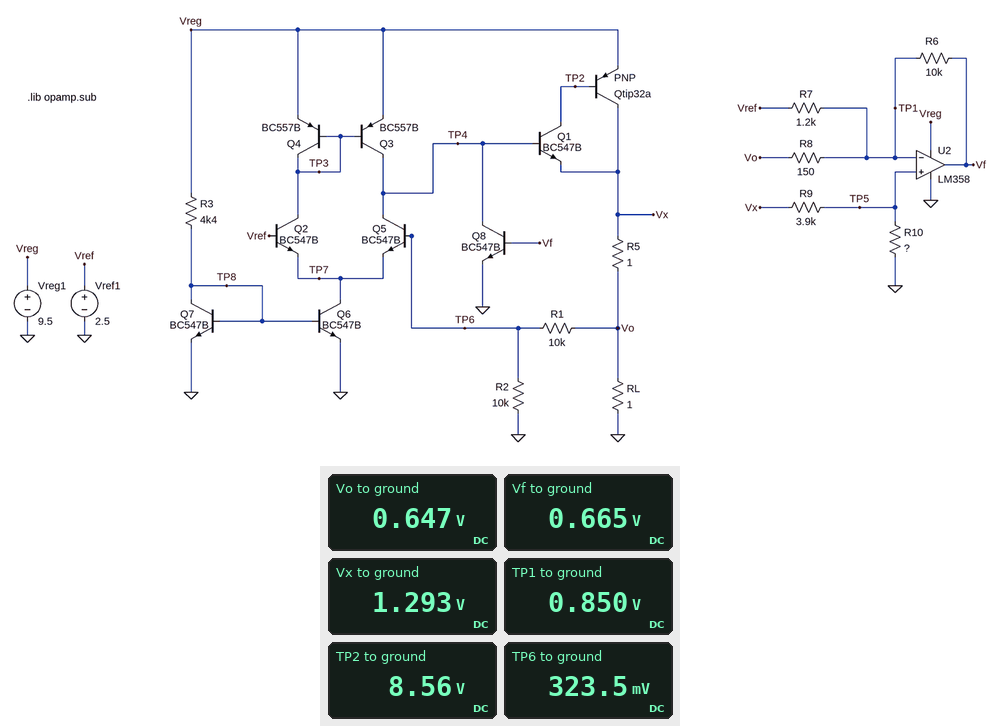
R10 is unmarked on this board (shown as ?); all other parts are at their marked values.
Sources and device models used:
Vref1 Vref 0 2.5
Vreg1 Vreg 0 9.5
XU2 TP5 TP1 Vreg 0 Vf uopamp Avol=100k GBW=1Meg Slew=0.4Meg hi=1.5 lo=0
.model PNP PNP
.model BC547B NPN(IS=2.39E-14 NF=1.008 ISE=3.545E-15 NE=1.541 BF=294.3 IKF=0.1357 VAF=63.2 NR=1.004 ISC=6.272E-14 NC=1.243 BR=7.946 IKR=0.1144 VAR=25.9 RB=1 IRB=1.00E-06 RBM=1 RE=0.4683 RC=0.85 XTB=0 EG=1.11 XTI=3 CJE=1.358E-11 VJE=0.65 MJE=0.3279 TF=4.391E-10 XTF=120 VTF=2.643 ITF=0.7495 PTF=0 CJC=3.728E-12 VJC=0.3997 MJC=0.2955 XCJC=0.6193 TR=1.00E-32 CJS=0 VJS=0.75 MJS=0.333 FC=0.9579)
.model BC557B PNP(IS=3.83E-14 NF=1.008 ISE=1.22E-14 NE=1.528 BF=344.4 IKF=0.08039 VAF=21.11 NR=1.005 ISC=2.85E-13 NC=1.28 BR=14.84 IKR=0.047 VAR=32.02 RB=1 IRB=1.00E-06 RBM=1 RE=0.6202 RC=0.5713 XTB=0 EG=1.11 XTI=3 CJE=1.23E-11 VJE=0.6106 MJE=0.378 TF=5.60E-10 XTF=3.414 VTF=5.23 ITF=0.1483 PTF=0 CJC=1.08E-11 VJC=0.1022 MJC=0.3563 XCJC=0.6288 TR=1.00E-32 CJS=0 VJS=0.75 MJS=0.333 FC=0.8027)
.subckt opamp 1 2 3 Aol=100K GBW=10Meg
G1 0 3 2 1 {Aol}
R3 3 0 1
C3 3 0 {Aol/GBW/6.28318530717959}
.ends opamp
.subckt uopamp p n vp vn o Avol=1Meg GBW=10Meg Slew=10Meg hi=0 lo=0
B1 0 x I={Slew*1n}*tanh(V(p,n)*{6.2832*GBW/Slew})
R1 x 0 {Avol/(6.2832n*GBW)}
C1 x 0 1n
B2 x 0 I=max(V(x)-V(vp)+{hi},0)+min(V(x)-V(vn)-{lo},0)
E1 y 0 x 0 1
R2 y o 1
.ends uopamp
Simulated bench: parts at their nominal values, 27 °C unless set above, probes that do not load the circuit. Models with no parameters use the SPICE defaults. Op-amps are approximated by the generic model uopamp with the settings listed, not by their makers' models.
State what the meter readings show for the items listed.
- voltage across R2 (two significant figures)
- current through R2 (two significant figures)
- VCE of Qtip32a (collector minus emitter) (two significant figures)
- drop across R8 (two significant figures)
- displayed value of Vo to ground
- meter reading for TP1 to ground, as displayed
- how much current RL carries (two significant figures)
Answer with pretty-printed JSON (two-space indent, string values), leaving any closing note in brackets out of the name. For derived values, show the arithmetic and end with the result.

{
  "voltage across R2": "323.5 mV = 320 mV",
  "current through R2": "(323.5 mV) / 10 kΩ = 32 µA",
  "VCE of Qtip32a (collector minus emitter)": "1.293 V - 9.5 V = -8.2 V",
  "drop across R8": "850 mV - 647 mV = 200 mV",
  "displayed value of Vo to ground": "0.647 V",
  "meter reading for TP1 to ground, as displayed": "0.850 V",
  "how much current RL carries": "(647 mV) / 1 Ω = 650 mA"
}
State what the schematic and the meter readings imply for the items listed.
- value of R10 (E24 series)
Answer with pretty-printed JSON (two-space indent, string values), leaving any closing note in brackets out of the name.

{
  "value of R10": "7.5 kΩ"
}
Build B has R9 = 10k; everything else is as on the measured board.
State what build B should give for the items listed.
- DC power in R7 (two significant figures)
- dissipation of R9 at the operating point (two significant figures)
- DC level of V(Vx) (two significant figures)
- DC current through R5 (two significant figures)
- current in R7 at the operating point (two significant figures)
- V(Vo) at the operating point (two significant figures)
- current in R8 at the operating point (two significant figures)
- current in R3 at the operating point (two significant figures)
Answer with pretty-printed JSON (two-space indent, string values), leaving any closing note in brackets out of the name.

{
  "DC power in R7": "1.8 mW",
  "dissipation of R9 at the operating point": "2.3 mW",
  "DC level of V(Vx)": "8.4 V",
  "DC current through R5": "4.2 A",
  "current in R7 at the operating point": "1.2 mA",
  "V(Vo) at the operating point": "4.2 V",
  "current in R8 at the operating point": "1.6 mA",
  "current in R3 at the operating point": "2.0 mA"
}
